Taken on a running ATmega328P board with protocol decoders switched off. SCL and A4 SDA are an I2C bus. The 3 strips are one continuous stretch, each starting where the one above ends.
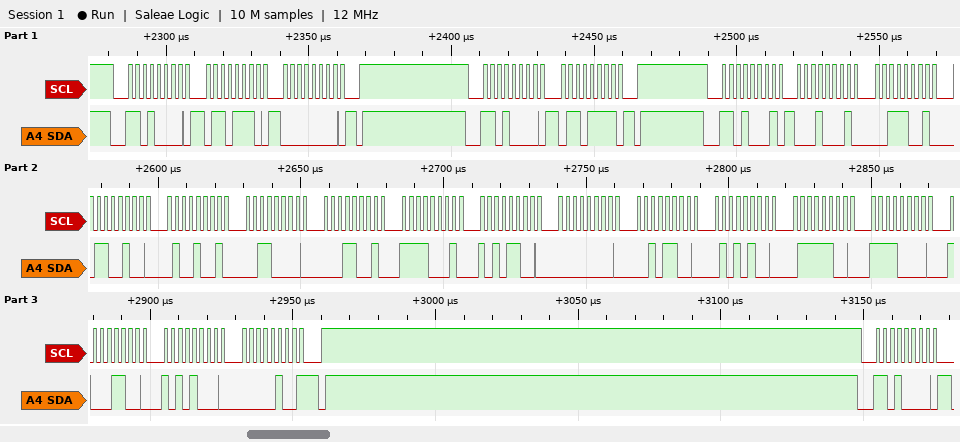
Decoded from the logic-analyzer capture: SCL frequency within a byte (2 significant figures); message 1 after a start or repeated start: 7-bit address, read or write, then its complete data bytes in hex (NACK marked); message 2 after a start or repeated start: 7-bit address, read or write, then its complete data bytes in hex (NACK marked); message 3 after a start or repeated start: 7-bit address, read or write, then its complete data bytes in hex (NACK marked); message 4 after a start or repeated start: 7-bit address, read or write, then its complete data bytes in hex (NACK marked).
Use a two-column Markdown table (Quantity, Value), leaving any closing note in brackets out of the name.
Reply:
| Quantity | Value |
|---|---|
| SCL frequency within a byte | 400 kHz |
| message 1 after a start or repeated start: 7-bit address, read or write, then its complete data bytes in hex | 0x68 write: 6E 00 |
| message 2 after a start or repeated start: 7-bit address, read or write, then its complete data bytes in hex | 0x68 write: 6F |
| message 3 after a start or repeated start: 7-bit address, read or write, then its complete data bytes in hex | 0x68 read: 11 39 64 49 30 19 F1 AC 00 2C 54 7C F0 8C A8 04 NACK |
| message 4 after a start or repeated start: 7-bit address, read or write, then its complete data bytes in hex | 0x68 write |
